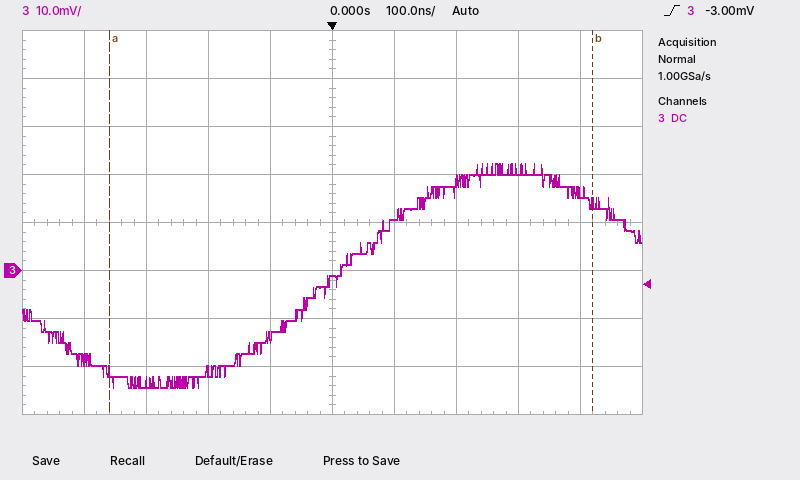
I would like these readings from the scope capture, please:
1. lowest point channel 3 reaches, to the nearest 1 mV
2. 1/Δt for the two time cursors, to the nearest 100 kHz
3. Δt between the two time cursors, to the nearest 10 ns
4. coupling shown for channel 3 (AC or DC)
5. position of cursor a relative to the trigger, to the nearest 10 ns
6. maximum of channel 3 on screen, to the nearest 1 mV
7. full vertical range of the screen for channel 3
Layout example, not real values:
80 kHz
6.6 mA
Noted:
-24 mV
1.3 MHz
780 ns
DC
-360 ns
22 mV
80 mV
